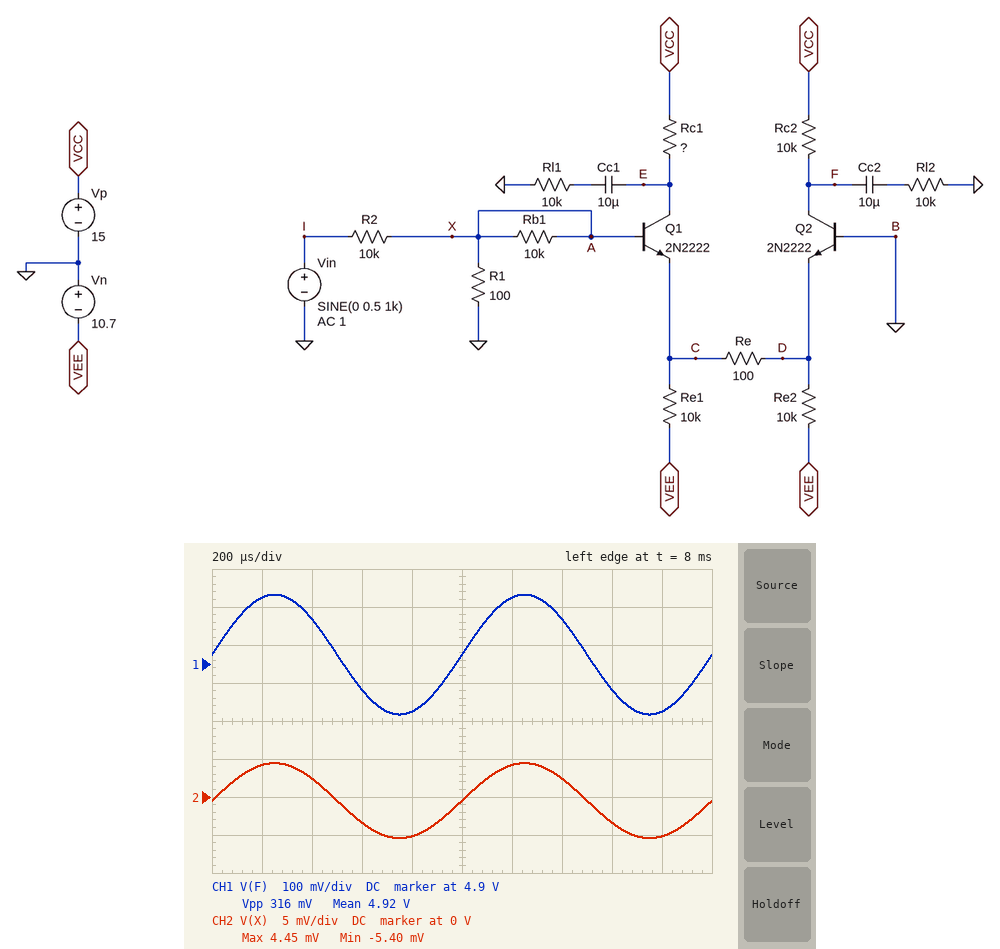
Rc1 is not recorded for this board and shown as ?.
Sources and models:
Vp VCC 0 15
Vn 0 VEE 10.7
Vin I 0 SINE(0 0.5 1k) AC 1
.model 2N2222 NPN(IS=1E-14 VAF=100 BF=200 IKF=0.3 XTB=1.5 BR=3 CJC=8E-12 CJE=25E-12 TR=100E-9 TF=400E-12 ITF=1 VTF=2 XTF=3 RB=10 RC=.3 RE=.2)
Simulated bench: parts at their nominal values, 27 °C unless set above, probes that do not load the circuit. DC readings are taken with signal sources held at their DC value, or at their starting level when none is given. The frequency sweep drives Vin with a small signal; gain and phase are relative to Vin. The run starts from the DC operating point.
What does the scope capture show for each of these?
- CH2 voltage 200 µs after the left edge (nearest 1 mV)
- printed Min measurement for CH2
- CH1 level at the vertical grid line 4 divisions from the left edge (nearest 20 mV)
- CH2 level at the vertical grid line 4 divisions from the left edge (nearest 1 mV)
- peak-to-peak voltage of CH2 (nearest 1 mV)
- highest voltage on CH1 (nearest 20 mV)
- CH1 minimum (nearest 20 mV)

4 mV
-5.40 mV
4.78 V
-5 mV
10 mV
5.08 V
4.76 V
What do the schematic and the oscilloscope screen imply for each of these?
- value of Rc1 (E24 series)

13 kΩ
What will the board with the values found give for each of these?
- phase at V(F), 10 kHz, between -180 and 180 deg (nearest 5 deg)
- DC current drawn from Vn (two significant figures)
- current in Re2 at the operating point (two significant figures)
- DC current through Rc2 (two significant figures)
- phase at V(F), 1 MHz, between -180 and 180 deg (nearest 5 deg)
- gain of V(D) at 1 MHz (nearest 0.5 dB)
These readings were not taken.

0 deg
2.0 mA
1.0 mA
1.0 mA
-15 deg
-55.5 dB
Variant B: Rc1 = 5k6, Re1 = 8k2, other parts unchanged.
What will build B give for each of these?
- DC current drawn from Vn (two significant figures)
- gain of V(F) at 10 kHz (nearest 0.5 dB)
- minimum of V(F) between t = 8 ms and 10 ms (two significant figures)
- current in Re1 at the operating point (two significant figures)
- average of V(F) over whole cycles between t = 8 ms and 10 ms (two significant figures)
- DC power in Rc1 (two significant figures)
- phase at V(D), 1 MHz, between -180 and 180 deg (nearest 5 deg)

2.2 mA
-9.5 dB
4.5 V
1.2 mA
4.7 V
7.9 mW
0 deg
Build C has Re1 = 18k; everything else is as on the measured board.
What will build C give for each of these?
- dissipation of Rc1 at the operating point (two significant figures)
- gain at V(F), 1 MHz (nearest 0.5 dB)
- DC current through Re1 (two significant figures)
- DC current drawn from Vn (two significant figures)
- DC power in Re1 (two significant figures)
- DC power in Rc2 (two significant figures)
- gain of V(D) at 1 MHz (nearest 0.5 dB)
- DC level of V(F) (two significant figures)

5.4 mW
-11.0 dB
560 µA
1.6 mA
5.6 mW
8.3 mW
-55.5 dB
5.9 V
